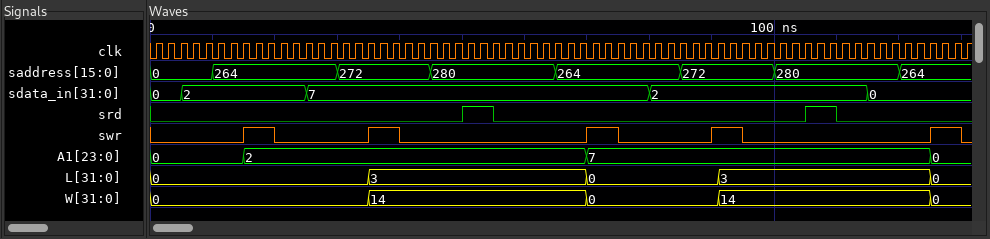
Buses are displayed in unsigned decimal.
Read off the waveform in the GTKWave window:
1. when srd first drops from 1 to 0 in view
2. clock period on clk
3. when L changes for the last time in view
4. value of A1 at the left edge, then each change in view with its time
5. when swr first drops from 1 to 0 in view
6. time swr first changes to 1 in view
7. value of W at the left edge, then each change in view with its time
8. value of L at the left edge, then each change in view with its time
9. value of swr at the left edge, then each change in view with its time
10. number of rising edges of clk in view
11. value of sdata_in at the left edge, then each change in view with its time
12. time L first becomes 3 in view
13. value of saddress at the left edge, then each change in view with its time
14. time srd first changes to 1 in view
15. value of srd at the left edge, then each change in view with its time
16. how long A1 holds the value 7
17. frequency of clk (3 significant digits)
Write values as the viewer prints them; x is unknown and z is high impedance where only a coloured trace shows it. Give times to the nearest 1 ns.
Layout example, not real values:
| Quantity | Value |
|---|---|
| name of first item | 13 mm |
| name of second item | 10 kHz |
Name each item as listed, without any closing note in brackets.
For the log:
| Quantity | Value |
|---|---|
| when srd first drops from 1 to 0 in view | 55 ns |
| clock period on clk | 2 ns |
| when L changes for the last time in view | 125 ns |
| value of A1 at the left edge, then each change in view with its time | 0, 2 at 15 ns, 7 at 70 ns, 0 at 125 ns |
| when swr first drops from 1 to 0 in view | 20 ns |
| time swr first changes to 1 in view | 15 ns |
| value of W at the left edge, then each change in view with its time | 0, 14 at 35 ns, 0 at 70 ns, 14 at 91 ns, 0 at 125 ns |
| value of L at the left edge, then each change in view with its time | 0, 3 at 35 ns, 0 at 70 ns, 3 at 91 ns, 0 at 125 ns |
| value of swr at the left edge, then each change in view with its time | 0, 1 at 15 ns, 0 at 20 ns, 1 at 35 ns, 0 at 40 ns, 1 at 70 ns, 0 at 75 ns, 1 at 90 ns, 0 at 95 ns, 1 at 125 ns, 0 at 130 ns |
| number of rising edges of clk in view | 66 |
| value of sdata_in at the left edge, then each change in view with its time | 0, 2 at 5 ns, 7 at 25 ns, 2 at 80 ns, 0 at 115 ns |
| time L first becomes 3 in view | 35 ns |
| value of saddress at the left edge, then each change in view with its time | 0, 264 at 10 ns, 272 at 30 ns, 280 at 45 ns, 264 at 65 ns, 272 at 85 ns, 280 at 100 ns, 264 at 120 ns |
| time srd first changes to 1 in view | 50 ns |
| value of srd at the left edge, then each change in view with its time | 0, 1 at 50 ns, 0 at 55 ns, 1 at 105 ns, 0 at 110 ns |
| how long A1 holds the value 7 | 55 ns |
| frequency of clk | 500 MHz |
